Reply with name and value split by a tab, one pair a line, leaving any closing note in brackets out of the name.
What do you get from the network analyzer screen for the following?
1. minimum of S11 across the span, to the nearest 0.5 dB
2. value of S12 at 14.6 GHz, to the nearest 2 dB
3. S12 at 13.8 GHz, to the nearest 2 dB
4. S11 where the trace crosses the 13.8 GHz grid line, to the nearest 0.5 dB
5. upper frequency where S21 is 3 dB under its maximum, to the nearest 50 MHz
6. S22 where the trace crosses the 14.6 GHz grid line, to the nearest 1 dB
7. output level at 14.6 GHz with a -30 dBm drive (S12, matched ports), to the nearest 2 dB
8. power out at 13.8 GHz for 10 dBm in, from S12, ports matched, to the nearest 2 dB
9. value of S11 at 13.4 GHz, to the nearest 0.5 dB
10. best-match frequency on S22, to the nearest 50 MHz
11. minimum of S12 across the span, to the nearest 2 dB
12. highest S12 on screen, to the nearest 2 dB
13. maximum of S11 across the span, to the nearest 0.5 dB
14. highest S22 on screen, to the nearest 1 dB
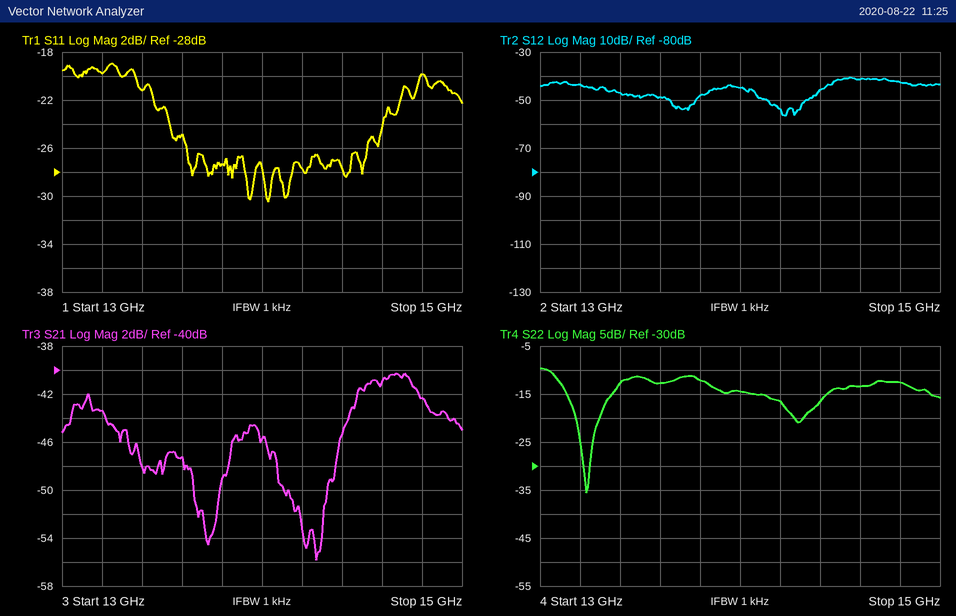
minimum of S11 across the span, to the nearest 0.5 dB	-30.5 dB
value of S12 at 14.6 GHz, to the nearest 2 dB	-42 dB
S12 at 13.8 GHz, to the nearest 2 dB	-48 dB
S11 where the trace crosses the 13.8 GHz grid line, to the nearest 0.5 dB	-27.5 dB
upper frequency where S21 is 3 dB under its maximum, to the nearest 50 MHz	14.85 GHz
S22 where the trace crosses the 14.6 GHz grid line, to the nearest 1 dB	-13 dB
output level at 14.6 GHz with a -30 dBm drive (S12, matched ports), to the nearest 2 dB	-72 dBm
power out at 13.8 GHz for 10 dBm in, from S12, ports matched, to the nearest 2 dB	-38 dBm
value of S11 at 13.4 GHz, to the nearest 0.5 dB	-21.0 dB
best-match frequency on S22, to the nearest 50 MHz	13.25 GHz
minimum of S12 across the span, to the nearest 2 dB	-56 dB
highest S12 on screen, to the nearest 2 dB	-40 dB
maximum of S11 across the span, to the nearest 0.5 dB	-19.0 dB
highest S22 on screen, to the nearest 1 dB	-10 dB
